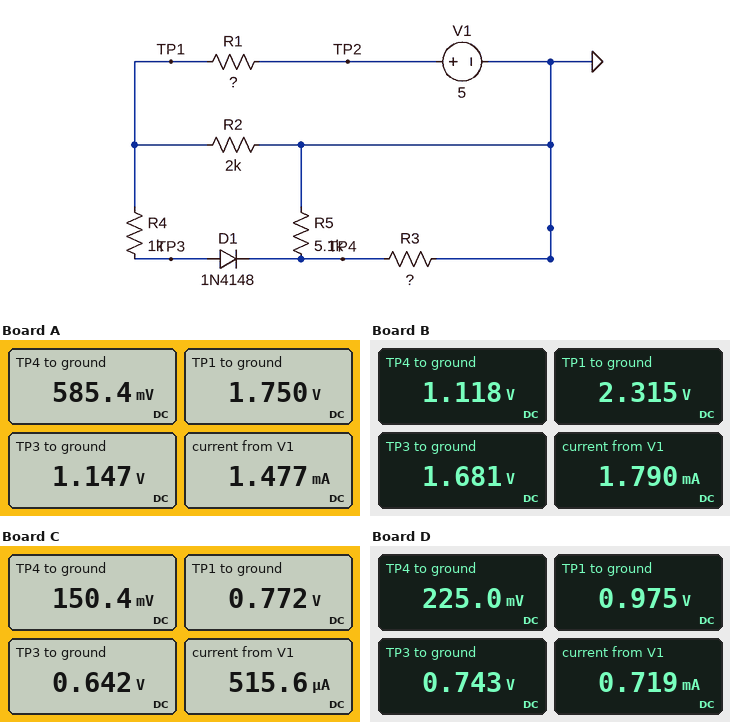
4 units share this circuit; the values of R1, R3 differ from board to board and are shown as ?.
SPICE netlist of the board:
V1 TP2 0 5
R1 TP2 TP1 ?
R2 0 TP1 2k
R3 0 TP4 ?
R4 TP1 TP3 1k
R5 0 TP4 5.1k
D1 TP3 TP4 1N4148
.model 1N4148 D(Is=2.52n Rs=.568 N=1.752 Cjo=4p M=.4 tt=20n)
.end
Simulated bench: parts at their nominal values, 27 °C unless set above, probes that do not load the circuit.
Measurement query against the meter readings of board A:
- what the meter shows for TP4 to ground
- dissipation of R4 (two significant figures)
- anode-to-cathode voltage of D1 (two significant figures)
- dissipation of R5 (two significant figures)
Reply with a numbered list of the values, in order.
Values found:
1. 585.4 mV
2. 360 µW
3. 560 mV
4. 67 µW
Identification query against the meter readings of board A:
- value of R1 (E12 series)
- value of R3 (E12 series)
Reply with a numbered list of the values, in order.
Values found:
1. 2.2 kΩ
2. 1.2 kΩ
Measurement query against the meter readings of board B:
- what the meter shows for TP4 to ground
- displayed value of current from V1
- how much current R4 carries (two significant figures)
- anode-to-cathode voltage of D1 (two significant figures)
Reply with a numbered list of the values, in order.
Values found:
1. 1.118 V
2. 1.790 mA
3. 630 µA
4. 560 mV
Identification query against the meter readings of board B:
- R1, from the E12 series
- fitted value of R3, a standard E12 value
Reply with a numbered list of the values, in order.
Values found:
1. 1.5 kΩ
2. 2.7 kΩ
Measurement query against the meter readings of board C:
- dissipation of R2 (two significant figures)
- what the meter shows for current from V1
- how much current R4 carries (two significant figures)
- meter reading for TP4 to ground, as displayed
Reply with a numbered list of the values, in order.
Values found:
1. 300 µW
2. 515.6 µA
3. 130 µA
4. 150.4 mV
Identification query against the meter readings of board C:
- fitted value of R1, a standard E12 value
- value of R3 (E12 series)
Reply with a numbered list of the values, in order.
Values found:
1. 8.2 kΩ
2. 1.5 kΩ
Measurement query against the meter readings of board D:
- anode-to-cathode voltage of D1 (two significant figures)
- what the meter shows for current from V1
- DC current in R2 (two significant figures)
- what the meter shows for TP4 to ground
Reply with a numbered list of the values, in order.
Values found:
1. 520 mV
2. 0.719 mA
3. 490 µA
4. 225.0 mV
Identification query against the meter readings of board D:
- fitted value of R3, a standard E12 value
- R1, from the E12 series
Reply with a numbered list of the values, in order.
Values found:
1. 1.2 kΩ
2. 5.6 kΩ
